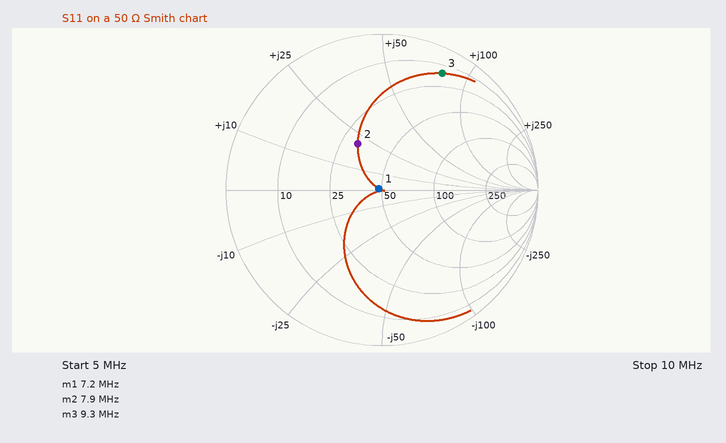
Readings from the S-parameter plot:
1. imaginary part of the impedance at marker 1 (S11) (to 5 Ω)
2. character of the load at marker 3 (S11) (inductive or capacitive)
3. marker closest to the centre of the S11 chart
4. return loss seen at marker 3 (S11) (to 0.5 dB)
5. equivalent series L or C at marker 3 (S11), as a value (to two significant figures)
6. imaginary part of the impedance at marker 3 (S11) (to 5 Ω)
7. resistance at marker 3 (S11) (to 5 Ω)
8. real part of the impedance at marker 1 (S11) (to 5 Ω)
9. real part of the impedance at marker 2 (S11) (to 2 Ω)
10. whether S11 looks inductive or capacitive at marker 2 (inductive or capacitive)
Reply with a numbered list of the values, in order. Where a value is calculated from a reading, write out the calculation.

1. 0 Ω
2. inductive
3. marker 1
4. 1.5 dB
5. L = 80 Ω/(2π × 9.3 MHz) ≈ 1.4 µH
6. +80 Ω
7. 15 Ω
8. 50 Ω
9. 32 Ω
10. inductive
